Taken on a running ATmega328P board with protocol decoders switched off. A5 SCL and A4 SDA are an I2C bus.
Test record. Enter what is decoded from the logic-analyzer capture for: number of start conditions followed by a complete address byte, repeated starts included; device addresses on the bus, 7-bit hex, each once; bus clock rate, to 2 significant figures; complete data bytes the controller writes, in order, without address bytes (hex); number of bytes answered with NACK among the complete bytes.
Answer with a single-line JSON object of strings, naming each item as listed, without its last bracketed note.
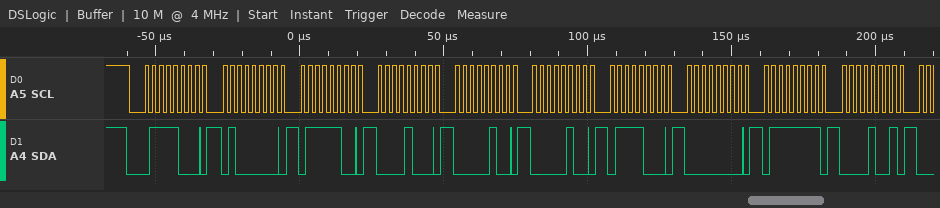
{"number of start conditions followed by a complete address byte, repeated starts included": "1", "device addresses on the bus, 7-bit hex, each once": "0x3C", "bus clock rate, to 2 significant figures": "400 kHz", "complete data bytes the controller writes, in order, without address bytes": "40 7C 08 04 04 78 00 7F 09", "number of bytes answered with NACK among the complete bytes": "0"}
